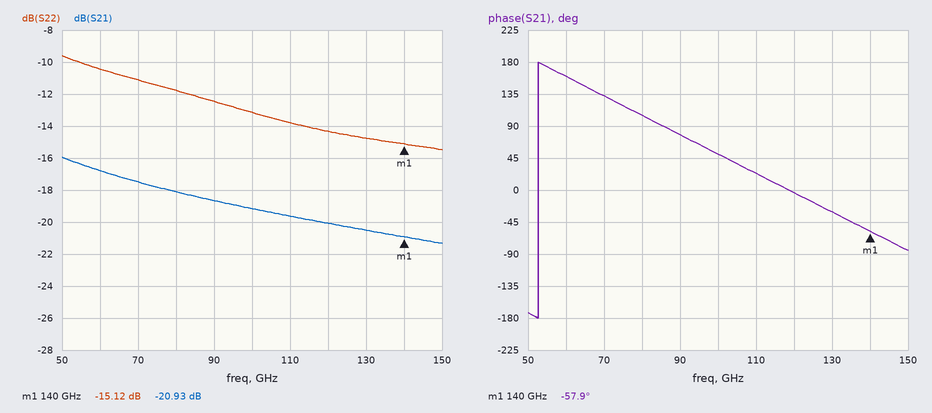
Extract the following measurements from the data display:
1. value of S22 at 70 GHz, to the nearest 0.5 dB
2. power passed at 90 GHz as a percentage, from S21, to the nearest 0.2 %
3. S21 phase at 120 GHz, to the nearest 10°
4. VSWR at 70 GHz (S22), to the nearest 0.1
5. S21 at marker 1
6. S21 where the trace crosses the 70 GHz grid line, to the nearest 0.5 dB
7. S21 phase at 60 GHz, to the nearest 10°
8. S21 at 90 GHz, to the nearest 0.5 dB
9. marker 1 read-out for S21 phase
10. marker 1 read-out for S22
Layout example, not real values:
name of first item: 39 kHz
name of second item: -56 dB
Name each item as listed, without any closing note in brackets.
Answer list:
value of S22 at 70 GHz, to the nearest 0.5 dB: -11.0 dB
power passed at 90 GHz as a percentage, from S21, to the nearest 0.2 %: 1.4 %
S21 phase at 120 GHz, to the nearest 10°: 0°
VSWR at 70 GHz (S22), to the nearest 0.1: 1.8
S21 at marker 1: -20.93 dB
S21 where the trace crosses the 70 GHz grid line, to the nearest 0.5 dB: -17.5 dB
S21 phase at 60 GHz, to the nearest 10°: 160°
S21 at 90 GHz, to the nearest 0.5 dB: -18.5 dB
marker 1 read-out for S21 phase: -57.9°
marker 1 read-out for S22: -15.12 dB
